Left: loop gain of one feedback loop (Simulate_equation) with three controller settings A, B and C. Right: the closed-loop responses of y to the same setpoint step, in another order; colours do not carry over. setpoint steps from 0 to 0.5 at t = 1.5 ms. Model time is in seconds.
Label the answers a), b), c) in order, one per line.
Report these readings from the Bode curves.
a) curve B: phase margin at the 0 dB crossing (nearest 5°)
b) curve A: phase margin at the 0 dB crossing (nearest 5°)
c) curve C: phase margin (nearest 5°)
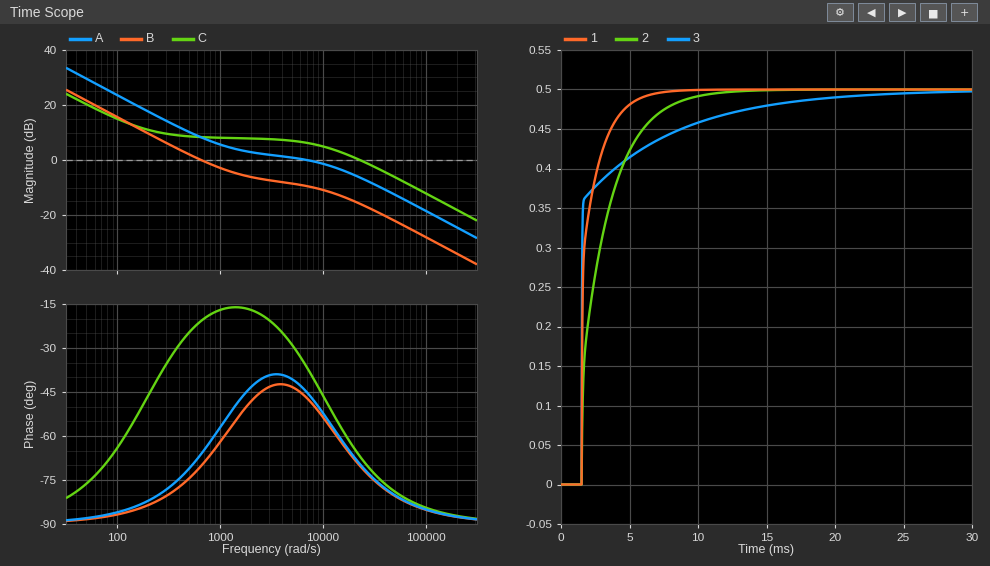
a) 110°
b) 135°
c) 115°
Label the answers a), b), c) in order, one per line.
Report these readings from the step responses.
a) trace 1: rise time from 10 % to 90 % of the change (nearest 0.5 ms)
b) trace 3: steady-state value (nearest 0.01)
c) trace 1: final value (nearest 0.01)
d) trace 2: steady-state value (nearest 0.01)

a) 2.0 ms
b) 0.50
c) 0.50
d) 0.50
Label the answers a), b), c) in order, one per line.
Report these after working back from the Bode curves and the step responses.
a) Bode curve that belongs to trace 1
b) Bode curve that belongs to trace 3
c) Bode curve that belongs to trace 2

a) A
b) C
c) B
